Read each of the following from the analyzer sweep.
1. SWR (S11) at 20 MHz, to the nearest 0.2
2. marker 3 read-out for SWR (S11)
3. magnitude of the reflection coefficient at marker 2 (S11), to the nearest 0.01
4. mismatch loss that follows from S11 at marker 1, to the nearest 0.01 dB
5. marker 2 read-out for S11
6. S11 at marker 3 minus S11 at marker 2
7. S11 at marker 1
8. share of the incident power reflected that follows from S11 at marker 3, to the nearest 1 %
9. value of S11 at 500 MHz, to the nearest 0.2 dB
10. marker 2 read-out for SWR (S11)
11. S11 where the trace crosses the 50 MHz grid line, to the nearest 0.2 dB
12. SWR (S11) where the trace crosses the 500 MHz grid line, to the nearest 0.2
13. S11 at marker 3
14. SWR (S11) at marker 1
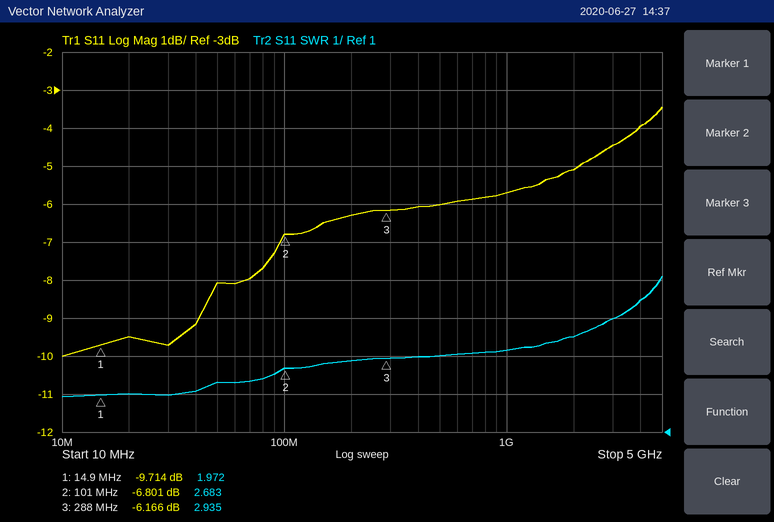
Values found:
2.0
2.935
0.46
0.49 dB
-6.801 dB
0.635 dB
-9.714 dB
24 %
-6.0 dB
2.683
-8.0 dB
3.0
-6.166 dB
1.972
